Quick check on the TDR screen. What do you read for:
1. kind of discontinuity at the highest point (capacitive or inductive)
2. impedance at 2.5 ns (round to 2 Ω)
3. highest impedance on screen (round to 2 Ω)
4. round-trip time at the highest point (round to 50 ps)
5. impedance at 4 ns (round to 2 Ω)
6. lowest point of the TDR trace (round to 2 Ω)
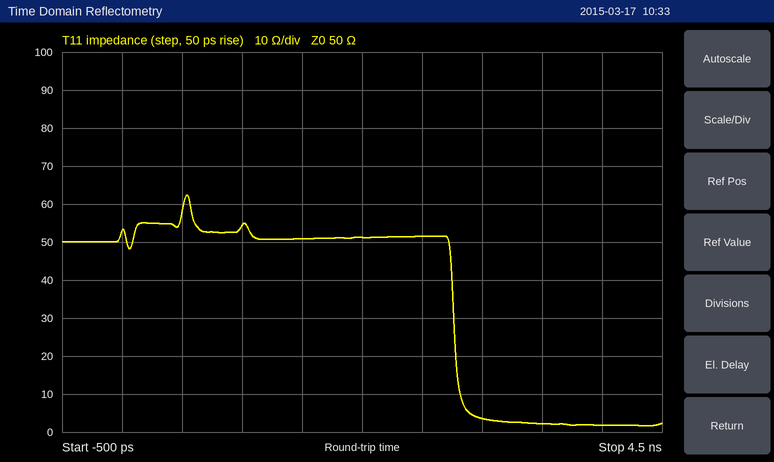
inductive
52 Ω
62 Ω
550 ps
2 Ω
2 Ω
